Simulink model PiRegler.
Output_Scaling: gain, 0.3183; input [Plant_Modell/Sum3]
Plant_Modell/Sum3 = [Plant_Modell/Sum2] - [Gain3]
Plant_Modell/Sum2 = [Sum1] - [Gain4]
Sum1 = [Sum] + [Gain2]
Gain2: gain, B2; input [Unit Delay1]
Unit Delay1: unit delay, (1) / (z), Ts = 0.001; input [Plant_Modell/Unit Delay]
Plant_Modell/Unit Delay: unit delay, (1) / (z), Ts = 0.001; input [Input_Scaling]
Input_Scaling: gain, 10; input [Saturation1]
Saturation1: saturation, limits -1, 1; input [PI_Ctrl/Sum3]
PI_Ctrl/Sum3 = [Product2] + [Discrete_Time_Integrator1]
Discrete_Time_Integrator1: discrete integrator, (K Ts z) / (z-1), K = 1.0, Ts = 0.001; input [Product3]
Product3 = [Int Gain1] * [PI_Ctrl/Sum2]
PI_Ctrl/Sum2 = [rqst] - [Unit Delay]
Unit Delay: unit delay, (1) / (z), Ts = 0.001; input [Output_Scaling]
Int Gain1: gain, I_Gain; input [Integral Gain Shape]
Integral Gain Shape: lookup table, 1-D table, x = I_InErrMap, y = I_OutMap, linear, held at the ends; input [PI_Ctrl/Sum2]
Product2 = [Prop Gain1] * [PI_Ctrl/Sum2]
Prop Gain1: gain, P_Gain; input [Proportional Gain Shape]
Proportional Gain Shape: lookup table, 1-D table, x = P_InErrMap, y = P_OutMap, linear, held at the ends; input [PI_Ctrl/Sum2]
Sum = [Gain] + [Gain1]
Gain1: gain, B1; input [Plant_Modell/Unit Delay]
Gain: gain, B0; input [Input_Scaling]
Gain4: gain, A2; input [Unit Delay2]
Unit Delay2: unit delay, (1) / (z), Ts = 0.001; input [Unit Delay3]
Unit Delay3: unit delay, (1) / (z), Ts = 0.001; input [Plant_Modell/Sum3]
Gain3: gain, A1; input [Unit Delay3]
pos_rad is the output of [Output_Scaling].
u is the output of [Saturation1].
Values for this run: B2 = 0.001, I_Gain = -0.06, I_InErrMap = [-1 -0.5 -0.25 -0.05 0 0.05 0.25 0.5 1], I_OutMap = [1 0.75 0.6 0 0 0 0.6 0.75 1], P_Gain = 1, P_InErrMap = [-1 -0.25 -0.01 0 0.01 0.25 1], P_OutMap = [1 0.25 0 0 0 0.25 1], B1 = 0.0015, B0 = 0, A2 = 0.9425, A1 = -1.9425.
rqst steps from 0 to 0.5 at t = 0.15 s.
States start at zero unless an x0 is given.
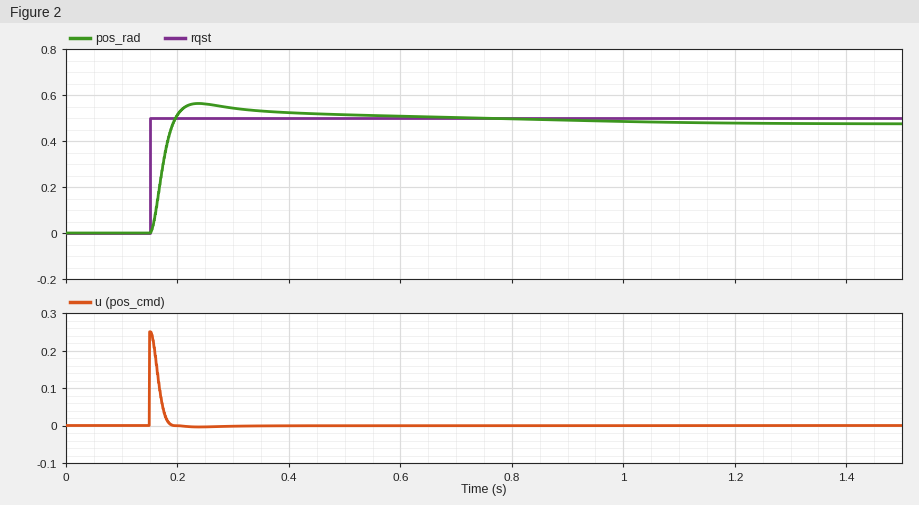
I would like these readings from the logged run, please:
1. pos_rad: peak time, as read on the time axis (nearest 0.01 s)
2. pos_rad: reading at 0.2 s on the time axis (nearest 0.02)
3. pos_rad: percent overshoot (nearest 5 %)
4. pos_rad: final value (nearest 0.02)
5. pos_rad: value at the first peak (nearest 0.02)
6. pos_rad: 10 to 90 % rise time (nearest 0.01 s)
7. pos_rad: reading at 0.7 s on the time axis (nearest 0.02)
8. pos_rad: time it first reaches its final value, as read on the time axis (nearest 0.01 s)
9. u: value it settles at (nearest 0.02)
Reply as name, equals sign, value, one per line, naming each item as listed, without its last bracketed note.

pos_rad: peak time, as read on the time axis = 0.24 s
pos_rad: reading at 0.2 s on the time axis = 0.52
pos_rad: percent overshoot = 20 %
pos_rad: final value = 0.48
pos_rad: value at the first peak = 0.56
pos_rad: 10 to 90 % rise time = 0.03 s
pos_rad: reading at 0.7 s on the time axis = 0.50
pos_rad: time it first reaches its final value, as read on the time axis = 0.19 s
u: value it settles at = 0.00
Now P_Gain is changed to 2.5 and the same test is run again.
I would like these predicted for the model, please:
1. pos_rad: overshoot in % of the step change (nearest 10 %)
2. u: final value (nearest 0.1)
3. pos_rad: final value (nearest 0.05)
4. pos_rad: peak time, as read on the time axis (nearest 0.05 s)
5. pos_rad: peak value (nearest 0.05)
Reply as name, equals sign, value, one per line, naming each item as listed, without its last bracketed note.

pos_rad: overshoot in % of the step change = 50 %
u: final value = 0.0
pos_rad: final value = 0.50
pos_rad: peak time, as read on the time axis = 0.20 s
pos_rad: peak value = 0.70
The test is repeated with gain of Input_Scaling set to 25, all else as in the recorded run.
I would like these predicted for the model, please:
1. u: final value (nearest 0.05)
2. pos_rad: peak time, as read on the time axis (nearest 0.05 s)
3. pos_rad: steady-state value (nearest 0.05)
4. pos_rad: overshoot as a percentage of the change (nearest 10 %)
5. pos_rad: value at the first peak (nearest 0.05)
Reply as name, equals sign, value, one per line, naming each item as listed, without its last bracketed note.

u: final value = 0.00
pos_rad: peak time, as read on the time axis = 0.20 s
pos_rad: steady-state value = 0.50
pos_rad: overshoot as a percentage of the change = 50 %
pos_rad: value at the first peak = 0.70
